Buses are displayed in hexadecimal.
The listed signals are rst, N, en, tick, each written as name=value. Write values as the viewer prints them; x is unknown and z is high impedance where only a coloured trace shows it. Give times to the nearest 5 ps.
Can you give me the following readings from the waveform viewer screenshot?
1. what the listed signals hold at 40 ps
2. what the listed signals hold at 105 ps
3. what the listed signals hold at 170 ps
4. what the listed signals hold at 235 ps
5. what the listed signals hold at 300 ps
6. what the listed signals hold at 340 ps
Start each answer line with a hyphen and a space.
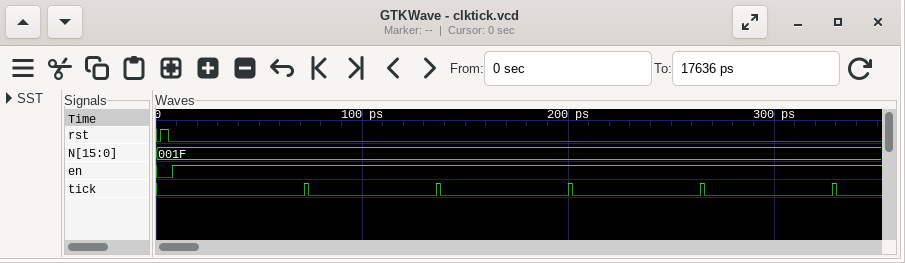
- rst=0, N=001F, en=1, tick=0
- rst=0, N=001F, en=1, tick=0
- rst=0, N=001F, en=1, tick=0
- rst=0, N=001F, en=1, tick=0
- rst=0, N=001F, en=1, tick=0
- rst=0, N=001F, en=1, tick=0
